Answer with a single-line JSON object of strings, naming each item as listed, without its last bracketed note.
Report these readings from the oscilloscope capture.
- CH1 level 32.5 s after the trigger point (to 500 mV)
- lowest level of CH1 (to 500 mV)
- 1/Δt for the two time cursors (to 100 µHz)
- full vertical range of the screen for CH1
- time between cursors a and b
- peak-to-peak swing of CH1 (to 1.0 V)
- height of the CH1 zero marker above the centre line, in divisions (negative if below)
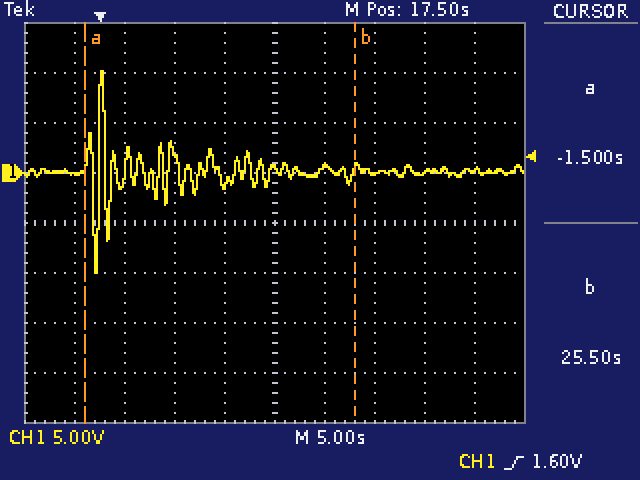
{"CH1 level 32.5 s after the trigger point": "0.0 V", "lowest level of CH1": "-10.0 V", "1/Δt for the two time cursors": "37.0 mHz", "full vertical range of the screen for CH1": "40 V", "time between cursors a and b": "27.0 s", "peak-to-peak swing of CH1": "20.0 V", "height of the CH1 zero marker above the centre line, in divisions": "+1.0 div"}
